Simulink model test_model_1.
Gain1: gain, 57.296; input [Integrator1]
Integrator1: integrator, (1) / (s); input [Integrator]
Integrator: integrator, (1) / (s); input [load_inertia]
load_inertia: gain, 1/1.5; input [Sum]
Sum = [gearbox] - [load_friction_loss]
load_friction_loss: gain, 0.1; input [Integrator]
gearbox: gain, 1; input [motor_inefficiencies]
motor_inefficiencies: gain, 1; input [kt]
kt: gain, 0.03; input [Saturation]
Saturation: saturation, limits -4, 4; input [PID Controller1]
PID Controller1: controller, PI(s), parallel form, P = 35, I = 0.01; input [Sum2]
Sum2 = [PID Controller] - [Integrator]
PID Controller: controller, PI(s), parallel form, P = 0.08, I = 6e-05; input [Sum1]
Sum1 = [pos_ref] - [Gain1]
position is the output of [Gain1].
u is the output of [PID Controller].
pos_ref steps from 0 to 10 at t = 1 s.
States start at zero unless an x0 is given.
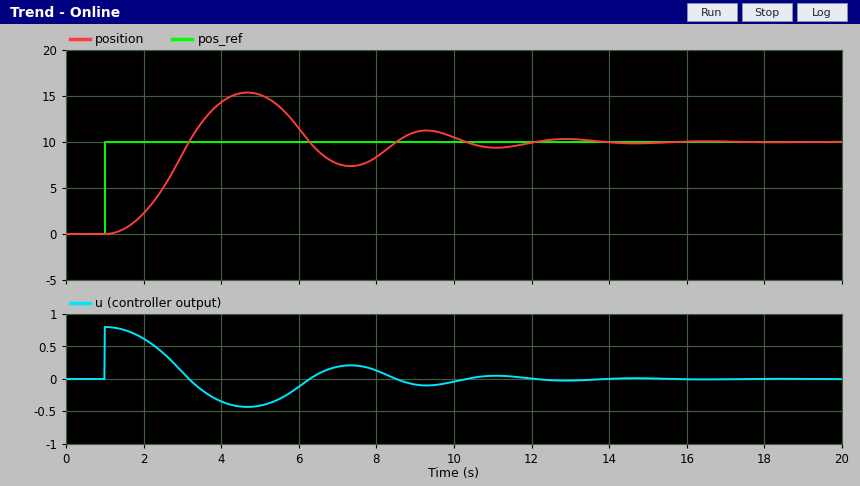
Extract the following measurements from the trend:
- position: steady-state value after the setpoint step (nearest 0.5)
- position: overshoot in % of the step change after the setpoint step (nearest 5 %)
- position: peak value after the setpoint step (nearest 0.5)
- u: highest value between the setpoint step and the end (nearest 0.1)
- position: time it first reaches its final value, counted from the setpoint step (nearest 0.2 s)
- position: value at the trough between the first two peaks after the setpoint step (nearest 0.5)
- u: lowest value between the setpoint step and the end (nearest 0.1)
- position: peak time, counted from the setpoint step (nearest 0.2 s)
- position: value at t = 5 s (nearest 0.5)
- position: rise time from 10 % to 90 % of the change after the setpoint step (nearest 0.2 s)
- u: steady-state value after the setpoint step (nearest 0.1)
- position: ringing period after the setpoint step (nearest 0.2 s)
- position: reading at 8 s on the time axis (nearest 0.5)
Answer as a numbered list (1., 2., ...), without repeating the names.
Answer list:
1. 10.0
2. 55 %
3. 15.5
4. 0.8
5. 2.2 s
6. 7.5
7. -0.4
8. 3.6 s
9. 15.0
10. 1.4 s
11. 0.0
12. 4.6 s
13. 8.5
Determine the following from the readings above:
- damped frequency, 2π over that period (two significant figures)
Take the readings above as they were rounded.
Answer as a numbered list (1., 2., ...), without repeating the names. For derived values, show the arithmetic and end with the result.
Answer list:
1. 2π / 4.6 = 1.4 rad/s
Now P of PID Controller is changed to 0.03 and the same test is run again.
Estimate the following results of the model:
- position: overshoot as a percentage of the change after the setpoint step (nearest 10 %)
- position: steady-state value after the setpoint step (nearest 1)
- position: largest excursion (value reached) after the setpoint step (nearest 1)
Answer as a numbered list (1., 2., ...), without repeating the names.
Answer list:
1. 30 %
2. 10
3. 13
